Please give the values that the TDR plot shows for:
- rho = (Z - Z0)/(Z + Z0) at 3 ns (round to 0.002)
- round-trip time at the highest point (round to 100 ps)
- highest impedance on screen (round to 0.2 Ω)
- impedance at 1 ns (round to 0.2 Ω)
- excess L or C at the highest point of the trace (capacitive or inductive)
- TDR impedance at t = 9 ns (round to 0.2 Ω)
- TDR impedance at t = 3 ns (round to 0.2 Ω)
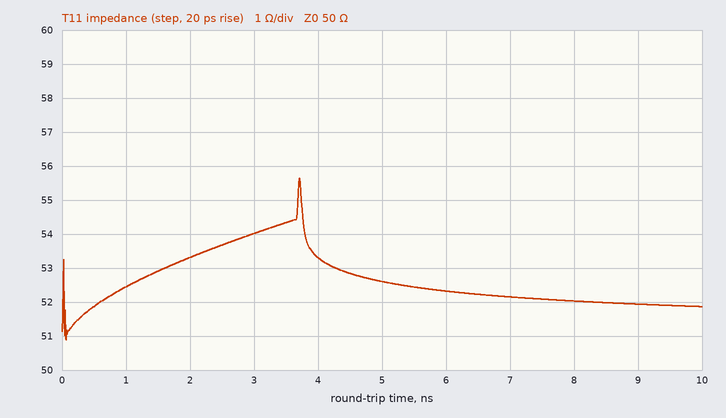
+0.038
3.7 ns
55.6 Ω
52.4 Ω
inductive
52.0 Ω
54.0 Ω
